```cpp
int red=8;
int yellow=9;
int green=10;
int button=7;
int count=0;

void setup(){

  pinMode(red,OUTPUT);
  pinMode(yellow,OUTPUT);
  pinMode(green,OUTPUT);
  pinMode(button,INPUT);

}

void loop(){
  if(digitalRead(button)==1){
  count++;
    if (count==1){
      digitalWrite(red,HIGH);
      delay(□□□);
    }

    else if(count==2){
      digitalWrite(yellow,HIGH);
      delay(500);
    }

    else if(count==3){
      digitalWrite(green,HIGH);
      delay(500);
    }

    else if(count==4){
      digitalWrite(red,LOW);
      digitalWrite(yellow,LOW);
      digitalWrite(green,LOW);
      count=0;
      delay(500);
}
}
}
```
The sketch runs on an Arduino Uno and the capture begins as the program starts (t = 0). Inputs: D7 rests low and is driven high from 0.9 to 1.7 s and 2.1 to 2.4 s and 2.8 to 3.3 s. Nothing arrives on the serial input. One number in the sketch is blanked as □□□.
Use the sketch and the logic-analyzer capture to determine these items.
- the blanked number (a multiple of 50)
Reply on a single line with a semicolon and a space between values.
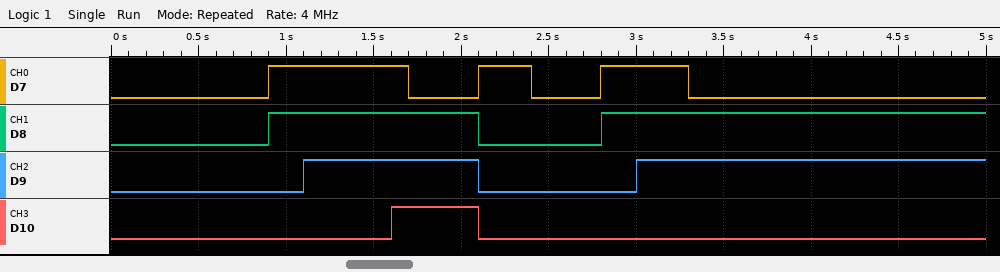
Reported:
200
